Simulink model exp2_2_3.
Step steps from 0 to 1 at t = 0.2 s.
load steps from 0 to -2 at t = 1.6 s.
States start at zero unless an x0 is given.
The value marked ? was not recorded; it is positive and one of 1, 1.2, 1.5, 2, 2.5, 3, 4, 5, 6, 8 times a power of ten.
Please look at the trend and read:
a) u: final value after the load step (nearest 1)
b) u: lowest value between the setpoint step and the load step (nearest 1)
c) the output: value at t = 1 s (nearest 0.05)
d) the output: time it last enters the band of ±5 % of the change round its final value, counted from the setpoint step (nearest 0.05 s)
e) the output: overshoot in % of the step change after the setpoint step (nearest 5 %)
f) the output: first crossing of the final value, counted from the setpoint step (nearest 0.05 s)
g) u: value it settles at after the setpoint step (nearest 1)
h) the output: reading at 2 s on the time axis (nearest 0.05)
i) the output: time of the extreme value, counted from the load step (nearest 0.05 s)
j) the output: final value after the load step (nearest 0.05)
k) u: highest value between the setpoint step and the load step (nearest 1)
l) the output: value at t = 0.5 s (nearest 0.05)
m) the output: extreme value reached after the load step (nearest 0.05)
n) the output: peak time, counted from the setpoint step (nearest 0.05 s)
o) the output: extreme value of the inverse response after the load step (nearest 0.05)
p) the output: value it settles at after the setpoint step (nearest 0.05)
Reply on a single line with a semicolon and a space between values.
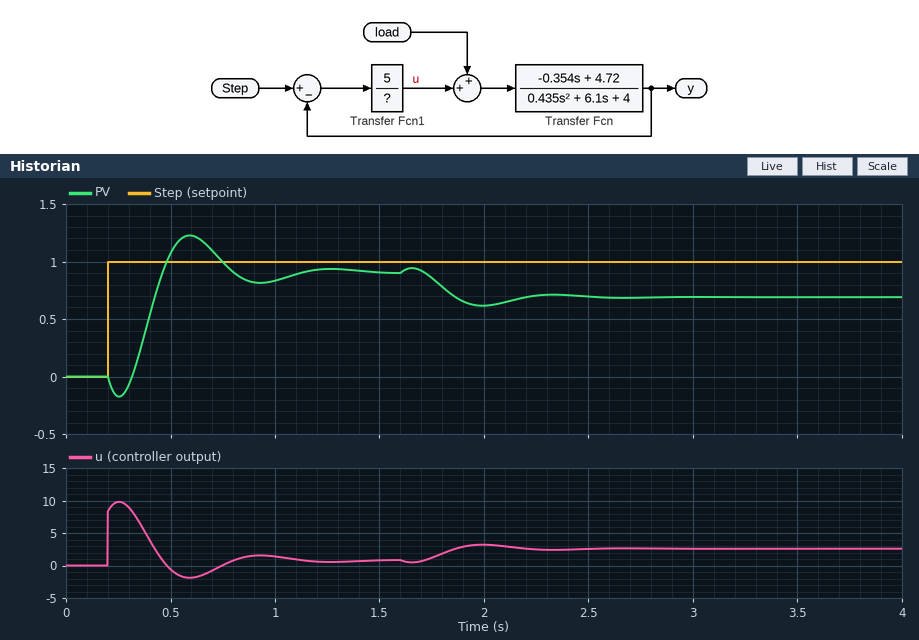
3; -2; 0.85; 0.85 s; 35 %; 0.25 s; 1; 0.60; 0.40 s; 0.70; 10; 1.05; 0.60; 0.40 s; 0.95; 0.90
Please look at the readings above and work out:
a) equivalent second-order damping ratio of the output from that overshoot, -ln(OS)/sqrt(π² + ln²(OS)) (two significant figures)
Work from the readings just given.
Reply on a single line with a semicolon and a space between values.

0.32
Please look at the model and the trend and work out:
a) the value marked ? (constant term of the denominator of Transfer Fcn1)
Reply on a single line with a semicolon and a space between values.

0.6
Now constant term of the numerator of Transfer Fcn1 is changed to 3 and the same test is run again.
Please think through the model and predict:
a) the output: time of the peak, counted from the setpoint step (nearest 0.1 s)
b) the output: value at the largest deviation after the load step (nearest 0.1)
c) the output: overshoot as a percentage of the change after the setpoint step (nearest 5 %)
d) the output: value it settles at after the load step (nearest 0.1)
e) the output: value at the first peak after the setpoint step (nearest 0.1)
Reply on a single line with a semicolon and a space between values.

0.6 s; 0.5; 10 %; 0.5; 0.9
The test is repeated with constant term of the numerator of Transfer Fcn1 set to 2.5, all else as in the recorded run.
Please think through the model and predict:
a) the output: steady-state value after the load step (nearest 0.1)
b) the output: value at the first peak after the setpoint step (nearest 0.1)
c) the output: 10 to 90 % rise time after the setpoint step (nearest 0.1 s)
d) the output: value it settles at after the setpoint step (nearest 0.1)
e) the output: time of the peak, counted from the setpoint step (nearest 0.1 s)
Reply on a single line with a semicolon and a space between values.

0.4; 0.9; 0.3 s; 0.8; 0.7 s
